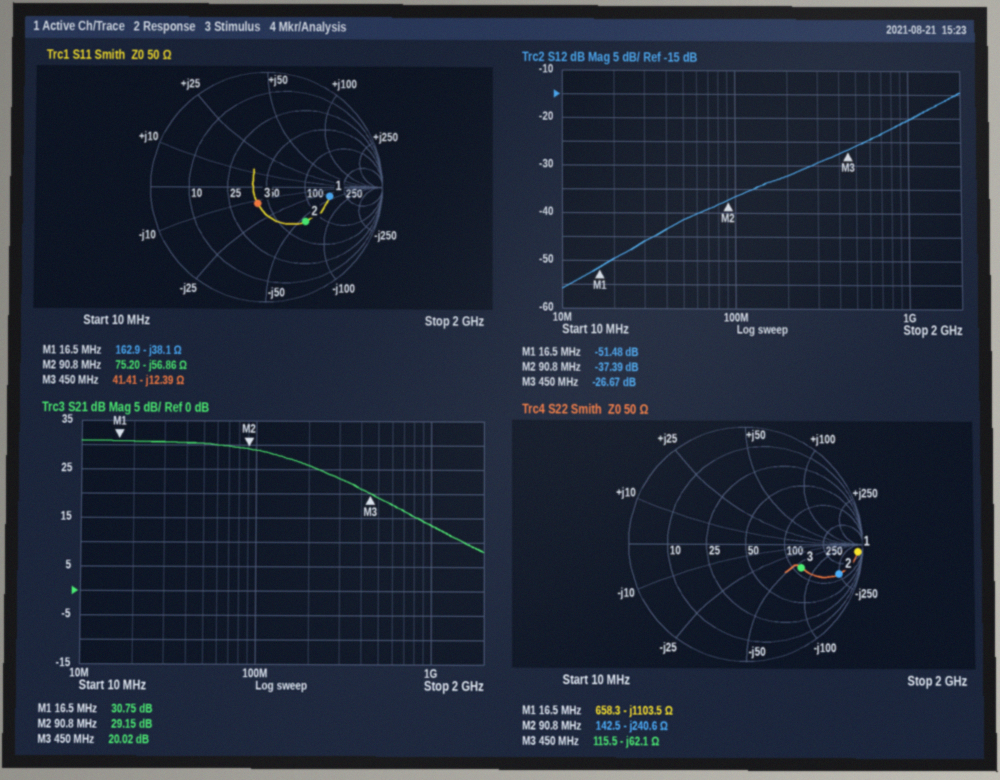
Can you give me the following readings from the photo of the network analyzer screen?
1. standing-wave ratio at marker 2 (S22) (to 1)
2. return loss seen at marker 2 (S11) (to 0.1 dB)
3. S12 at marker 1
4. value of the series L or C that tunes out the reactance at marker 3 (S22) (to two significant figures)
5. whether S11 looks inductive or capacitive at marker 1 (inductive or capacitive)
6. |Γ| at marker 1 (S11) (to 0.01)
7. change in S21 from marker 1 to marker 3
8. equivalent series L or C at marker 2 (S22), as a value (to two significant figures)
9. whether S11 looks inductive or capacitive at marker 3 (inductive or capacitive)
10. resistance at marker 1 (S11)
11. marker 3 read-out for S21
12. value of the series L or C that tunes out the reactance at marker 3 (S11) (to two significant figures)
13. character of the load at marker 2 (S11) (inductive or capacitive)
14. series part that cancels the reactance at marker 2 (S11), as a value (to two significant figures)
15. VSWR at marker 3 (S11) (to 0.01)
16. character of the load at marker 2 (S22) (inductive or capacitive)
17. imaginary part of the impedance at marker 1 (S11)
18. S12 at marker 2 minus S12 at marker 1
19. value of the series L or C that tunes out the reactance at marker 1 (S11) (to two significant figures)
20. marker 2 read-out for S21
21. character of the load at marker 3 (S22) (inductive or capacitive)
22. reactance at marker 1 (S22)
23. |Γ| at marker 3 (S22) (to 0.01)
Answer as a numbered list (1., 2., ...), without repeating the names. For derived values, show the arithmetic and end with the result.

1. 11
2. 6.9 dB
3. -51.48 dB
4. L = 62.1 Ω/(2π × 450 MHz) ≈ 22 nH
5. capacitive
6. 0.55
7. 20.02 − (30.75) = -10.73 dB
8. C = 1/(2π × 90.8 MHz × 240.6 Ω) ≈ 7.3 pF
9. capacitive
10. 162.9 Ω
11. 20.02 dB
12. L = 12.39 Ω/(2π × 450 MHz) ≈ 4.4 nH
13. capacitive
14. L = 56.86 Ω/(2π × 90.8 MHz) ≈ 100 nH
15. 1.39
16. capacitive
17. -38.1 Ω
18. -37.39 − (-51.48) = 14.09 dB
19. L = 38.1 Ω/(2π × 16.5 MHz) ≈ 368 nH, so 370 nH to two significant figures
20. 29.15 dB
21. capacitive
22. -1103.5 Ω
23. 0.51
